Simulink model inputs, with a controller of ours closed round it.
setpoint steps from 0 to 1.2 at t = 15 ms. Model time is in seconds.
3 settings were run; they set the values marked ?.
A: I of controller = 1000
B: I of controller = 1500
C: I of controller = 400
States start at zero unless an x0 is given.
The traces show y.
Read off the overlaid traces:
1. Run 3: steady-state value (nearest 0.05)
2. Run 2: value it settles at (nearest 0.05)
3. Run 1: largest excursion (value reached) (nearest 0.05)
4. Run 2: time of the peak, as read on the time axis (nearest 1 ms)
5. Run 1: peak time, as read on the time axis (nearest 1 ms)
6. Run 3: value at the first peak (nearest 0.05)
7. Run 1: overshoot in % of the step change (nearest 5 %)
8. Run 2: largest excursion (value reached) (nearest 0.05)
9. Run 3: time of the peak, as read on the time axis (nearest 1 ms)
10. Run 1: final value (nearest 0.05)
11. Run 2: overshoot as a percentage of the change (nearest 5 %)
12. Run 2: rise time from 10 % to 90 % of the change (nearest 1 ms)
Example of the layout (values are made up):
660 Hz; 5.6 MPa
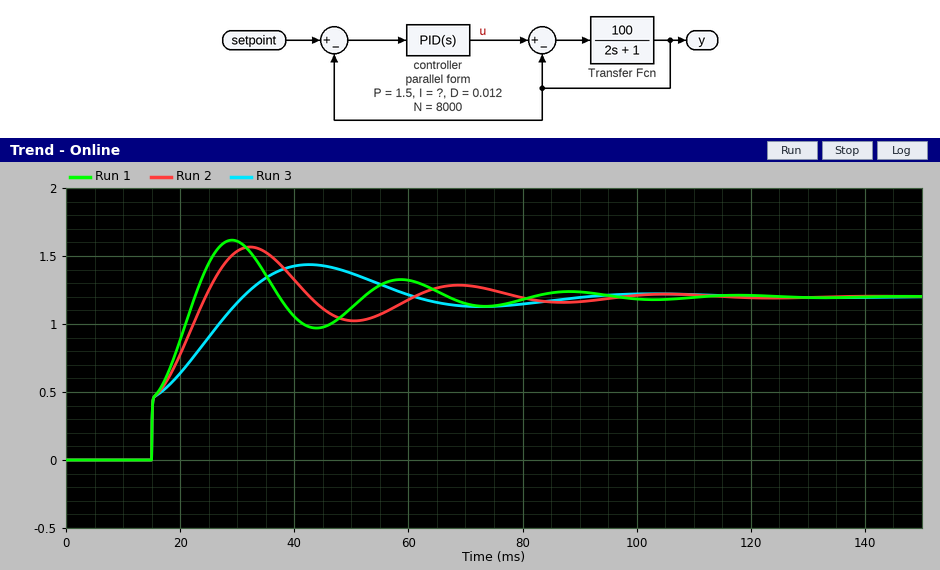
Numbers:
1.20; 1.20; 1.60; 32 ms; 29 ms; 1.45; 35 %; 1.55; 43 ms; 1.20; 30 %; 8 ms
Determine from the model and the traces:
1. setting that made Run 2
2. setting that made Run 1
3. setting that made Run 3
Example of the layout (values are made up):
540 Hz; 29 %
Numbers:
A; B; C
